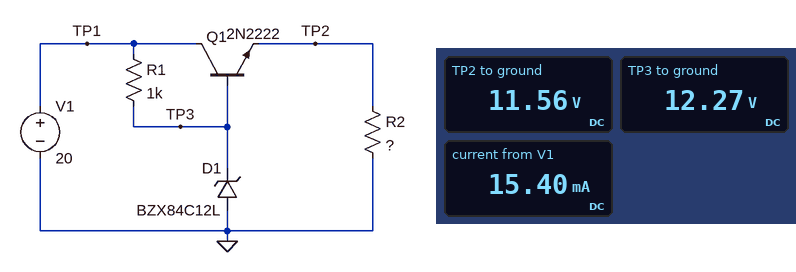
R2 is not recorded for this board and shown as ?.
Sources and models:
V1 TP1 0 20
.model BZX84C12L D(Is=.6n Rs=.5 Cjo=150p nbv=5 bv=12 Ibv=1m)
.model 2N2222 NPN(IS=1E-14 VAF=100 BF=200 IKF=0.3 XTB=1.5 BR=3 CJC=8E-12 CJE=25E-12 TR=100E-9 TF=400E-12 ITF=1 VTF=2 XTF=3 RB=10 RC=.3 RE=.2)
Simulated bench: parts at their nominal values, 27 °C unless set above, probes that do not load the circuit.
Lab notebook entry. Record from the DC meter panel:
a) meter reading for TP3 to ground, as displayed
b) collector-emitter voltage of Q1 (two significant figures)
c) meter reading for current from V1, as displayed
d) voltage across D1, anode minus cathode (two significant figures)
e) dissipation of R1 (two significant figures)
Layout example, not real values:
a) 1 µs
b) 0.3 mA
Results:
a) 12.27 V
b) 8.4 V
c) 15.40 mA
d) -12 V
e) 60 mW
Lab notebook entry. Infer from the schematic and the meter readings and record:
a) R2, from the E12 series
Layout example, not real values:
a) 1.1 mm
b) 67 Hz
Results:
a) 1.5 kΩ
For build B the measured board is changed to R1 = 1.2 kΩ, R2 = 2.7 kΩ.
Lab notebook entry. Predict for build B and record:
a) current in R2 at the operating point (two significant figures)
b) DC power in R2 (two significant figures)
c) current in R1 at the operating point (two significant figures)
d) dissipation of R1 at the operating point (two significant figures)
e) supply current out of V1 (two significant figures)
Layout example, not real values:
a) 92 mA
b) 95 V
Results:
a) 4.3 mA
b) 49 mW
c) 6.5 mA
d) 50 mW
e) 11 mA
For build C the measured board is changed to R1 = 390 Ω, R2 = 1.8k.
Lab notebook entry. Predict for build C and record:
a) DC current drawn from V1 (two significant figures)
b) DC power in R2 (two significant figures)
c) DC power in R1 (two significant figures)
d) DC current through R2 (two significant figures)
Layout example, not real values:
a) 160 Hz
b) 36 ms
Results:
a) 26 mA
b) 76 mW
c) 150 mW
d) 6.5 mA
